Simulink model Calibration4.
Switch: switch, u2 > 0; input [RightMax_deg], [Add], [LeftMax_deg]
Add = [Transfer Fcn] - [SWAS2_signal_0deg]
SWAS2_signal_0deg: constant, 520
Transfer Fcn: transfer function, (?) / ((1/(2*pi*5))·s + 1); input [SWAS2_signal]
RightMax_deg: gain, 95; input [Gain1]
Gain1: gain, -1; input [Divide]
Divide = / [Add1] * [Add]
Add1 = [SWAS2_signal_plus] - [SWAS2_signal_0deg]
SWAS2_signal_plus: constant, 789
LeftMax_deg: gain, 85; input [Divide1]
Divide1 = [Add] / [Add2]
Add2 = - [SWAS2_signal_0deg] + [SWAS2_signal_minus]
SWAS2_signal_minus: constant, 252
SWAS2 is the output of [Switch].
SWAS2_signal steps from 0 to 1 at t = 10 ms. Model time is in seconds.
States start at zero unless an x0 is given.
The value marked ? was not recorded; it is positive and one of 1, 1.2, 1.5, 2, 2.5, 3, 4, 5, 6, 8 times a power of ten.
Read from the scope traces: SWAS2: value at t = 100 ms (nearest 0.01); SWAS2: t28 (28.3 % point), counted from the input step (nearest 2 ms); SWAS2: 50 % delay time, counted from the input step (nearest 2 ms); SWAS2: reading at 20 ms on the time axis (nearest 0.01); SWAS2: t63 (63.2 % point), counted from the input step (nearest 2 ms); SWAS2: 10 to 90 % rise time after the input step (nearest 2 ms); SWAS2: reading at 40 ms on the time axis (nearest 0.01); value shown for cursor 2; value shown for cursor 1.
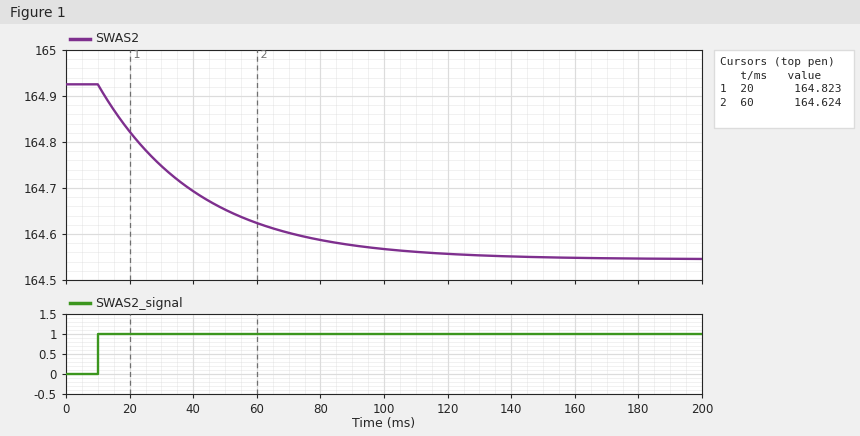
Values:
164.57
10 ms
22 ms
164.82
32 ms
70 ms
164.69
164.624
164.823
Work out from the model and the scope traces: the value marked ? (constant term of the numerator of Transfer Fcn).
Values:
1.2
